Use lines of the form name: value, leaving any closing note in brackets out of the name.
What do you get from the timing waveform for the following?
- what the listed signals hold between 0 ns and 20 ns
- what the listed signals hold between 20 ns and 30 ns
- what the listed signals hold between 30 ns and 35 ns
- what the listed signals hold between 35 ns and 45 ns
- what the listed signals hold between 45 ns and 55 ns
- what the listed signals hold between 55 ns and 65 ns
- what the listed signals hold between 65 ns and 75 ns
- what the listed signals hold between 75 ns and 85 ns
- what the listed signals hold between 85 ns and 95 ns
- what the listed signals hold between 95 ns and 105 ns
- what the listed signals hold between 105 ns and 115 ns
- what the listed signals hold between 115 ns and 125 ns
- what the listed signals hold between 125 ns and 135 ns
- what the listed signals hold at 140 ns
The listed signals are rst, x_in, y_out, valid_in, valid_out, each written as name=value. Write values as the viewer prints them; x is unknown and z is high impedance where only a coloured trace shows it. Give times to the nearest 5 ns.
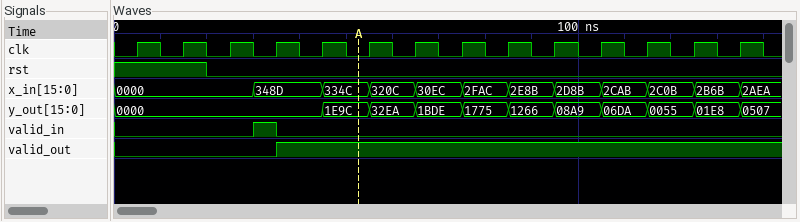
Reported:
what the listed signals hold between 0 ns and 20 ns: rst=1, x_in=0000, y_out=0000, valid_in=0, valid_out=0
what the listed signals hold between 20 ns and 30 ns: rst=0, x_in=0000, y_out=0000, valid_in=0, valid_out=0
what the listed signals hold between 30 ns and 35 ns: rst=0, x_in=348D, y_out=0000, valid_in=1, valid_out=0
what the listed signals hold between 35 ns and 45 ns: rst=0, x_in=348D, y_out=0000, valid_in=0, valid_out=1
what the listed signals hold between 45 ns and 55 ns: rst=0, x_in=334C, y_out=1E9C, valid_in=0, valid_out=1
what the listed signals hold between 55 ns and 65 ns: rst=0, x_in=320C, y_out=32EA, valid_in=0, valid_out=1
what the listed signals hold between 65 ns and 75 ns: rst=0, x_in=30EC, y_out=1BDE, valid_in=0, valid_out=1
what the listed signals hold between 75 ns and 85 ns: rst=0, x_in=2FAC, y_out=1775, valid_in=0, valid_out=1
what the listed signals hold between 85 ns and 95 ns: rst=0, x_in=2E8B, y_out=1266, valid_in=0, valid_out=1
what the listed signals hold between 95 ns and 105 ns: rst=0, x_in=2D8B, y_out=08A9, valid_in=0, valid_out=1
what the listed signals hold between 105 ns and 115 ns: rst=0, x_in=2CAB, y_out=06DA, valid_in=0, valid_out=1
what the listed signals hold between 115 ns and 125 ns: rst=0, x_in=2C0B, y_out=0055, valid_in=0, valid_out=1
what the listed signals hold between 125 ns and 135 ns: rst=0, x_in=2B6B, y_out=01E8, valid_in=0, valid_out=1
what the listed signals hold at 140 ns: rst=0, x_in=2AEA, y_out=0507, valid_in=0, valid_out=1
